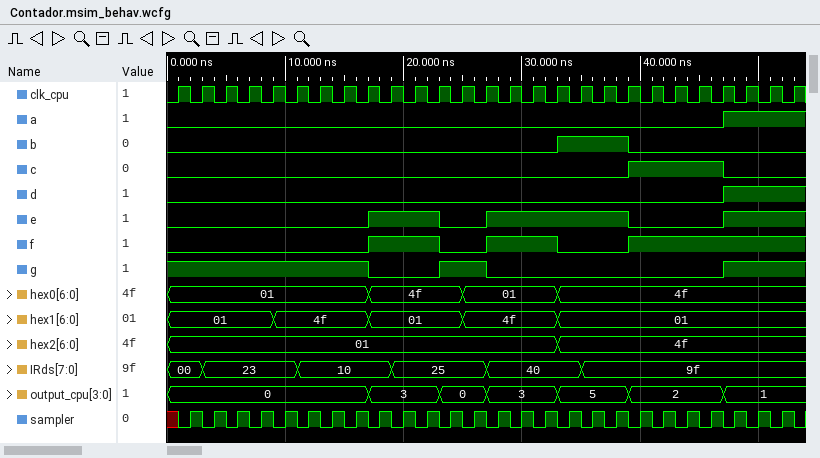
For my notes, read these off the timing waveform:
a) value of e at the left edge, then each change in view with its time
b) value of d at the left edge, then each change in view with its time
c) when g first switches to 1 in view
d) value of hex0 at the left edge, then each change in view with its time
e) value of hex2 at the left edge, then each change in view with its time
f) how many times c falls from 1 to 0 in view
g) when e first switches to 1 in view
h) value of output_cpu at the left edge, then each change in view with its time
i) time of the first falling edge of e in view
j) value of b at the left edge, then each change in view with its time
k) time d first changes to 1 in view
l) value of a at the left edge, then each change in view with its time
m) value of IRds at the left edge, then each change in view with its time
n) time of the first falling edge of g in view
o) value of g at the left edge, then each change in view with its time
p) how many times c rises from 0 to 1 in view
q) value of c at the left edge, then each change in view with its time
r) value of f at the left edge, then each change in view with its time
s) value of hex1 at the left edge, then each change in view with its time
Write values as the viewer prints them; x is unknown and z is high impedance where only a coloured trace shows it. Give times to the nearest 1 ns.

0, 1 at 17 ns, 0 at 23 ns, 1 at 27 ns, 0 at 39 ns, 1 at 47 ns
0, 1 at 47 ns
23 ns
01, 4f at 17 ns, 01 at 25 ns, 4f at 33 ns
01, 4f at 33 ns
1
17 ns
0, 3 at 17 ns, 0 at 23 ns, 3 at 27 ns, 5 at 33 ns, 2 at 39 ns, 1 at 47 ns
23 ns
0, 1 at 33 ns, 0 at 39 ns
47 ns
0, 1 at 47 ns
00, 23 at 3 ns, 10 at 11 ns, 25 at 19 ns, 40 at 27 ns, 9f at 35 ns
17 ns
1, 0 at 17 ns, 1 at 23 ns, 0 at 27 ns, 1 at 47 ns
1
0, 1 at 39 ns, 0 at 47 ns
0, 1 at 17 ns, 0 at 23 ns, 1 at 27 ns, 0 at 33 ns, 1 at 39 ns
01, 4f at 9 ns, 01 at 17 ns, 4f at 25 ns, 01 at 33 ns
